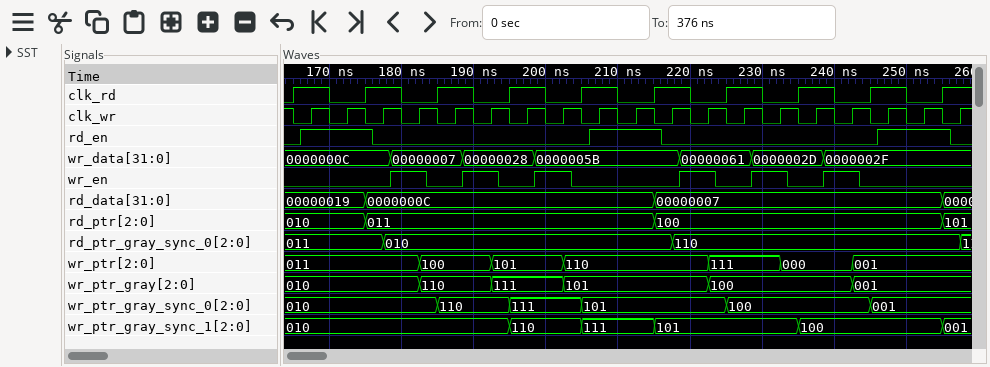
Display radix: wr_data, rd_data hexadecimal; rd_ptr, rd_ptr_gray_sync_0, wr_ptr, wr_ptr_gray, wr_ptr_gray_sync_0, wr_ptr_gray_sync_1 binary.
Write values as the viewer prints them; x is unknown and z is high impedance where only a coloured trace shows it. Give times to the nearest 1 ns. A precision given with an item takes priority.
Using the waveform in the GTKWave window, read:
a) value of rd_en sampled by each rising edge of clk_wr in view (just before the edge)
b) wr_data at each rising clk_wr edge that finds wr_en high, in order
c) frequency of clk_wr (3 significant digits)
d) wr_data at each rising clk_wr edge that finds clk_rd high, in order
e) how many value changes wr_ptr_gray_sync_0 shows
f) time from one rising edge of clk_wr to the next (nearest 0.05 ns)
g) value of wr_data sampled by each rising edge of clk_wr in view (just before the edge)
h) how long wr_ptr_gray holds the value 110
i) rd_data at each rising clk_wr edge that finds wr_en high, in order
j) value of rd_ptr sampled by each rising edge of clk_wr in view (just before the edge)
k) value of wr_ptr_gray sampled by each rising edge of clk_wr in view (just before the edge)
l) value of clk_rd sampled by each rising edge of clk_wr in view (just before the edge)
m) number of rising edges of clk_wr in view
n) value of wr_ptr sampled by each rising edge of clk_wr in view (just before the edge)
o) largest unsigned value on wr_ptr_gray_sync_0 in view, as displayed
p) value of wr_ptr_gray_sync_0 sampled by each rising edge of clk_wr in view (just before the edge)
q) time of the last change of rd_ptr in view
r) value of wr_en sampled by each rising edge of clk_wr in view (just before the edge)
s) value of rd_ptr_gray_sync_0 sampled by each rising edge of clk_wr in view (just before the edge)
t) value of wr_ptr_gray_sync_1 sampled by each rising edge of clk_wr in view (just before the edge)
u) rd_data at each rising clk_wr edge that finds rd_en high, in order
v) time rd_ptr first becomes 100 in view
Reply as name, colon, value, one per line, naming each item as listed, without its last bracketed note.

value of rd_en sampled by each rising edge of clk_wr in view: 1 1 0 0 0 0 0 0 1 1 0 0 0 0 0 0 1 1 0
wr_data at each rising clk_wr edge that finds wr_en high, in order: 00000007, 00000028, 0000005B, 00000061, 0000002D, 0000002F
frequency of clk_wr: 200 MHz
wr_data at each rising clk_wr edge that finds clk_rd high, in order: 0000000C, 0000000C, 00000007, 00000028, 0000005B, 0000005B, 00000061, 0000002D, 0000002F, 0000002F
how many value changes wr_ptr_gray_sync_0 shows: 5
time from one rising edge of clk_wr to the next: 5 ns
value of wr_data sampled by each rising edge of clk_wr in view: 0000000C, 0000000C, 0000000C, 00000007, 00000007, 00000028, 00000028, 0000005B, 0000005B, 0000005B, 0000005B, 00000061, 00000061, 0000002D, 0000002D, 0000002F, 0000002F, 0000002F, 0000002F
how long wr_ptr_gray holds the value 110: 10 ns
rd_data at each rising clk_wr edge that finds wr_en high, in order: 0000000C, 0000000C, 0000000C, 00000007, 00000007, 00000007
value of rd_ptr sampled by each rising edge of clk_wr in view: 010, 010, 011, 011, 011, 011, 011, 011, 011, 011, 100, 100, 100, 100, 100, 100, 100, 100, 101
value of wr_ptr_gray sampled by each rising edge of clk_wr in view: 010, 010, 010, 010, 110, 110, 111, 111, 101, 101, 101, 101, 100, 100, 100, 100, 001, 001, 001
value of clk_rd sampled by each rising edge of clk_wr in view: 1 0 1 0 1 0 1 0 1 0 1 0 1 0 1 0 1 0 1
number of rising edges of clk_wr in view: 19
value of wr_ptr sampled by each rising edge of clk_wr in view: 011, 011, 011, 011, 100, 100, 101, 101, 110, 110, 110, 110, 111, 111, 000, 000, 001, 001, 001
largest unsigned value on wr_ptr_gray_sync_0 in view, as displayed: 111
value of wr_ptr_gray_sync_0 sampled by each rising edge of clk_wr in view: 010, 010, 010, 010, 110, 110, 111, 111, 101, 101, 101, 101, 100, 100, 100, 100, 001, 001, 001
time of the last change of rd_ptr in view: 255 ns
value of wr_en sampled by each rising edge of clk_wr in view: 0 0 0 1 0 1 0 1 0 0 0 1 0 1 0 1 0 0 0
value of rd_ptr_gray_sync_0 sampled by each rising edge of clk_wr in view: 011, 011, 011, 010, 010, 010, 010, 010, 010, 010, 010, 110, 110, 110, 110, 110, 110, 110, 110
value of wr_ptr_gray_sync_1 sampled by each rising edge of clk_wr in view: 010, 010, 010, 010, 010, 010, 110, 110, 111, 111, 101, 101, 101, 101, 100, 100, 100, 100, 001
rd_data at each rising clk_wr edge that finds rd_en high, in order: 00000019, 00000019, 0000000C, 0000000C, 00000007, 00000007
time rd_ptr first becomes 100 in view: 215 ns
